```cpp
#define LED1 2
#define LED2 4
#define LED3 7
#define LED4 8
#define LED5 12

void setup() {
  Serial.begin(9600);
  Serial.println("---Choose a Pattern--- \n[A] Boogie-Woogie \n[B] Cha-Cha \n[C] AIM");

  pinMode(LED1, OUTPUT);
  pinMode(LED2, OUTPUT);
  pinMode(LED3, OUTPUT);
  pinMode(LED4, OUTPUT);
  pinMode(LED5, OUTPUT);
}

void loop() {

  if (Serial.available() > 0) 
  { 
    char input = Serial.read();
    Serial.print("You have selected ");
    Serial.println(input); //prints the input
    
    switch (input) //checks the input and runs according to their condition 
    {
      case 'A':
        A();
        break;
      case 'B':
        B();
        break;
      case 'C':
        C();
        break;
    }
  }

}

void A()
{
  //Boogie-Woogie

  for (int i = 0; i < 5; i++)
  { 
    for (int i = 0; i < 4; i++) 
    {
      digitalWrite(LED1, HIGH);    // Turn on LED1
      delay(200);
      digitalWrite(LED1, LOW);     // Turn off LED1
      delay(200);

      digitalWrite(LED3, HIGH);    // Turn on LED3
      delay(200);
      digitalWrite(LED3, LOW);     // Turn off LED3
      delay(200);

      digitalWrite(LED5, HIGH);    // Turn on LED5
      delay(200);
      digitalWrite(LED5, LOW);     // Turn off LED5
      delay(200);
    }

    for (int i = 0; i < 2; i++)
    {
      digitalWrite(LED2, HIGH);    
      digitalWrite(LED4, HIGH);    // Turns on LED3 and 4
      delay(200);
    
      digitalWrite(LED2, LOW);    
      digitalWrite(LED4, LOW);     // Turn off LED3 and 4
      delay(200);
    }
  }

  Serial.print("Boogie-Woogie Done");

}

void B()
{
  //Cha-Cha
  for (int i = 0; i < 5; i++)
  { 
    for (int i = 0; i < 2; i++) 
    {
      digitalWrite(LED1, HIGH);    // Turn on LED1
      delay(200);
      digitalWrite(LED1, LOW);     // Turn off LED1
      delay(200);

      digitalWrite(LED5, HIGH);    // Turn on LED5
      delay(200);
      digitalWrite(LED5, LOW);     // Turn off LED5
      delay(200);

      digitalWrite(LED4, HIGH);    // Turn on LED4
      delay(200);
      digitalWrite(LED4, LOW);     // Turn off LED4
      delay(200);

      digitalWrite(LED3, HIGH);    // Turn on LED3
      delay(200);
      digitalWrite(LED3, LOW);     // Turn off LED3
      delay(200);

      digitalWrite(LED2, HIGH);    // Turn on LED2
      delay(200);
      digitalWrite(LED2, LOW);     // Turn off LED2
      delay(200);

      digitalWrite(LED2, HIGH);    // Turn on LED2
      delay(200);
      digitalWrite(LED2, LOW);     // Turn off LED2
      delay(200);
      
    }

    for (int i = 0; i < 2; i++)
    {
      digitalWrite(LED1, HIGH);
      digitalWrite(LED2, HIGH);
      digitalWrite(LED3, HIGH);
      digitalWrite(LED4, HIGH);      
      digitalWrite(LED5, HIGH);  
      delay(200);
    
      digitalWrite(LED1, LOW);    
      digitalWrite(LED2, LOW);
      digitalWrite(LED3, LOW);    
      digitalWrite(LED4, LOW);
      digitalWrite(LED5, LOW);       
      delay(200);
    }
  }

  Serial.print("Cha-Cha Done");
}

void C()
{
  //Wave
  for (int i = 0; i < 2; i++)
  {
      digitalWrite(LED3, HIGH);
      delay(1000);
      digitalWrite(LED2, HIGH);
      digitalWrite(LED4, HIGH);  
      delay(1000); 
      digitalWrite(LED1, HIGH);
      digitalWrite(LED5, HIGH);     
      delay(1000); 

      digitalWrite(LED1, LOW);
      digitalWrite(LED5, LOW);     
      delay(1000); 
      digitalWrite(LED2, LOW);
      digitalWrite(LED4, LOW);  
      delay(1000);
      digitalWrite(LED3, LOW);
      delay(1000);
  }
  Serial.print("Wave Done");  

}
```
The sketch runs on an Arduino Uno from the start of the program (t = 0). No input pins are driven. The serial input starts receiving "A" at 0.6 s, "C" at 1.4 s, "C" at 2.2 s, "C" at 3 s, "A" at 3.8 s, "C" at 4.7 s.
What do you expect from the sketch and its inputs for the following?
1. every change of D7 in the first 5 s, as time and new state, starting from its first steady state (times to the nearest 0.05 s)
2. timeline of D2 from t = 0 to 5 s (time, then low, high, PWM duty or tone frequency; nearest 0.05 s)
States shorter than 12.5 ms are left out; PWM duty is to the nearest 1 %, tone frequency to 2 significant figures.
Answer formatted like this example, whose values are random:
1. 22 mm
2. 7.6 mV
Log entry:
1. 0 s low; 1 s high; 1.2 s low; 2.2 s high; 2.4 s low; 3.4 s high; 3.6 s low; 4.6 s high; 4.8 s low
2. 0 s low; 0.6 s high; 0.8 s low; 1.8 s high; 2 s low; 3 s high; 3.2 s low; 4.2 s high; 4.4 s low
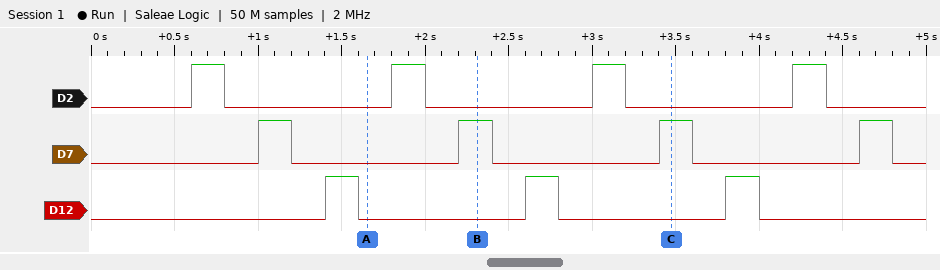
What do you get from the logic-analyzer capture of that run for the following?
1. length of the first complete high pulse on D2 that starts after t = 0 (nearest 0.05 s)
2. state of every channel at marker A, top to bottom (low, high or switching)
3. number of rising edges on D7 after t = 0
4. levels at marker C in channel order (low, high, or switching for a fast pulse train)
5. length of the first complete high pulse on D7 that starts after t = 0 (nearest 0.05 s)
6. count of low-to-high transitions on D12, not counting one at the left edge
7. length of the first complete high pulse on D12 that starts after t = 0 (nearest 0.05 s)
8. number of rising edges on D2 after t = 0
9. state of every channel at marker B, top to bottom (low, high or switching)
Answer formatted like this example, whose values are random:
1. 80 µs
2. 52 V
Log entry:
1. 0.20 s
2. D2 low, D7 low, D12 low
3. 4
4. D2 low, D7 high, D12 low
5. 0.20 s
6. 3
7. 0.20 s
8. 4
9. D2 low, D7 high, D12 low
